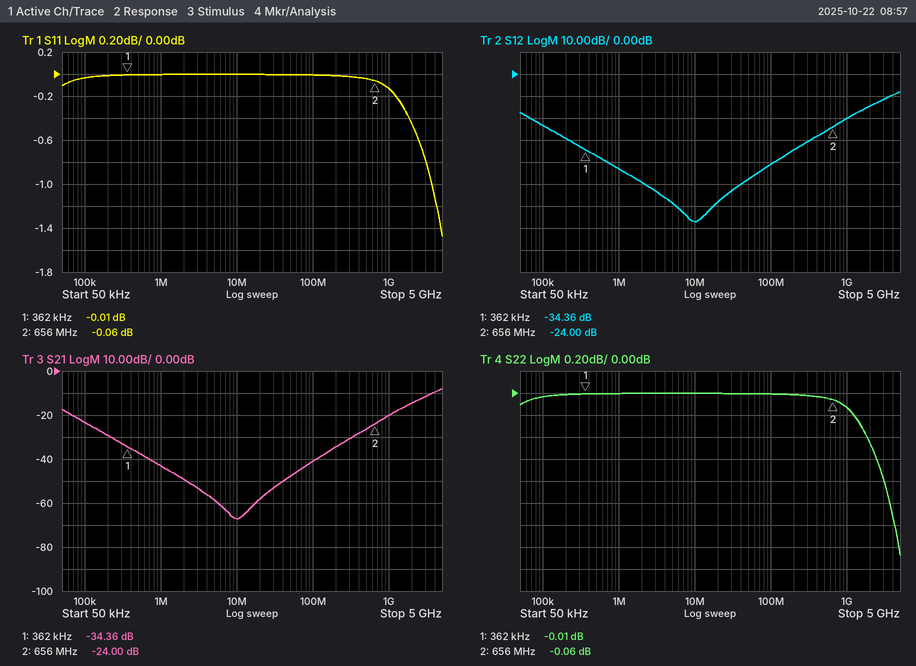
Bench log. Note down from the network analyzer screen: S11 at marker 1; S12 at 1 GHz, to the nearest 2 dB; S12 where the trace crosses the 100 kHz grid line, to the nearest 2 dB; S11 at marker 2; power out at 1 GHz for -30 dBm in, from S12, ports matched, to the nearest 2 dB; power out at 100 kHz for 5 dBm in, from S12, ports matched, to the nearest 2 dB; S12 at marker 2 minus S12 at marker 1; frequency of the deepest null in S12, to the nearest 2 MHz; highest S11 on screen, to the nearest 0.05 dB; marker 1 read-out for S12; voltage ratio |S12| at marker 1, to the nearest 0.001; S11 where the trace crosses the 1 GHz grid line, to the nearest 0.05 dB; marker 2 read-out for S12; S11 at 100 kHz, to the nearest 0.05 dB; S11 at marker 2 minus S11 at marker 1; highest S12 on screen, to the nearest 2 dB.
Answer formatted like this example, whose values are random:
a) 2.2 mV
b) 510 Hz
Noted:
a) -0.01 dB
b) -20 dB
c) -24 dB
d) -0.06 dB
e) -50 dBm
f) -18 dBm
g) 10.36 dB
h) 10 MHz
i) 0.00 dB
j) -34.36 dB
k) 0.019
l) -0.15 dB
m) -24.00 dB
n) -0.05 dB
o) -0.05 dB
p) -8 dB
